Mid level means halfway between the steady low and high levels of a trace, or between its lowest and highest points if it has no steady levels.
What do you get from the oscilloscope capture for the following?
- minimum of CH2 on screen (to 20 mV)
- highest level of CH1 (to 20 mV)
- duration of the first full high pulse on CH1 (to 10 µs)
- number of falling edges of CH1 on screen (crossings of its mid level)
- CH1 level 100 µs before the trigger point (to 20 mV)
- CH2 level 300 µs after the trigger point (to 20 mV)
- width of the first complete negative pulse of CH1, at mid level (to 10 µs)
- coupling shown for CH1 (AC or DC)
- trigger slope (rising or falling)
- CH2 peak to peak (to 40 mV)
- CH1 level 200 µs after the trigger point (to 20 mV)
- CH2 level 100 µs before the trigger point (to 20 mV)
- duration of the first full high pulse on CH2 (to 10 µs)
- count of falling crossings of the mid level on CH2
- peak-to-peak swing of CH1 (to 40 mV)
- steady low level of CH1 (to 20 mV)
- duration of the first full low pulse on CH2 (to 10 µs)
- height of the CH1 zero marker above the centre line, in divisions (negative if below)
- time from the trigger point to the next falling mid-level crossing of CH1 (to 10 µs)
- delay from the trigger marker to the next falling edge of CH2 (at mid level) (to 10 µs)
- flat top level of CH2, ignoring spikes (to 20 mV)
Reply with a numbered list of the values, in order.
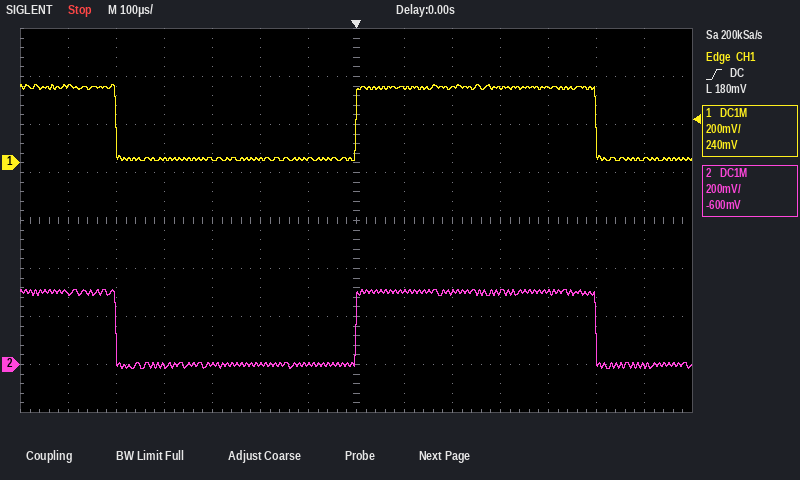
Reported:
1. -20 mV
2. 320 mV
3. 500 µs
4. 2
5. 20 mV
6. 300 mV
7. 500 µs
8. DC
9. rising
10. 320 mV
11. 320 mV
12. 0 mV
13. 500 µs
14. 2
15. 320 mV
16. 20 mV
17. 500 µs
18. +1.2 div
19. 500 µs
20. 500 µs
21. 300 mV
